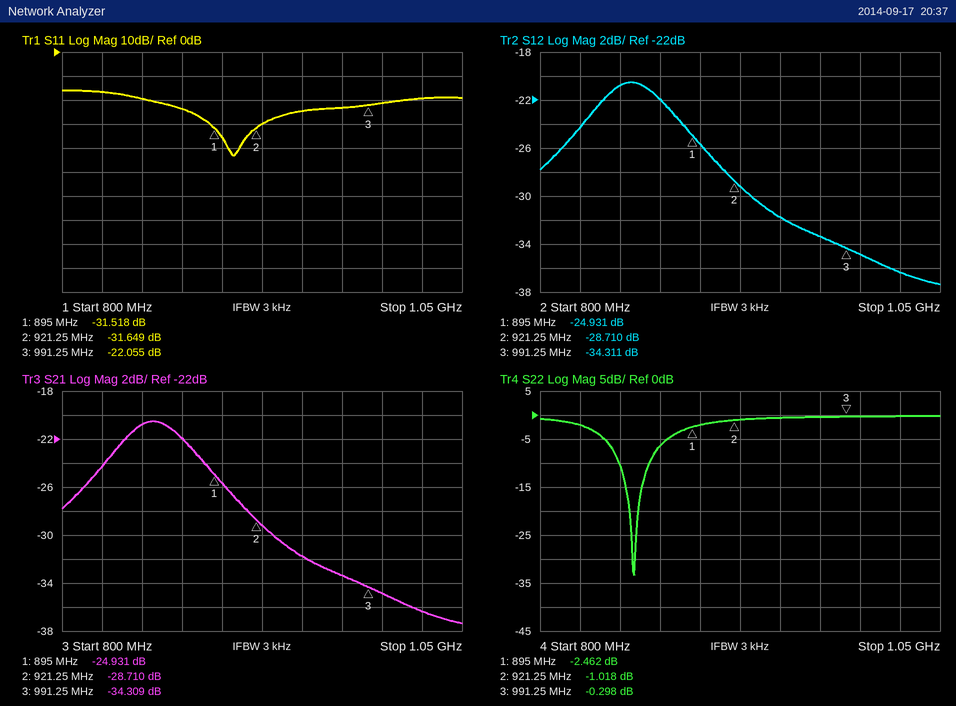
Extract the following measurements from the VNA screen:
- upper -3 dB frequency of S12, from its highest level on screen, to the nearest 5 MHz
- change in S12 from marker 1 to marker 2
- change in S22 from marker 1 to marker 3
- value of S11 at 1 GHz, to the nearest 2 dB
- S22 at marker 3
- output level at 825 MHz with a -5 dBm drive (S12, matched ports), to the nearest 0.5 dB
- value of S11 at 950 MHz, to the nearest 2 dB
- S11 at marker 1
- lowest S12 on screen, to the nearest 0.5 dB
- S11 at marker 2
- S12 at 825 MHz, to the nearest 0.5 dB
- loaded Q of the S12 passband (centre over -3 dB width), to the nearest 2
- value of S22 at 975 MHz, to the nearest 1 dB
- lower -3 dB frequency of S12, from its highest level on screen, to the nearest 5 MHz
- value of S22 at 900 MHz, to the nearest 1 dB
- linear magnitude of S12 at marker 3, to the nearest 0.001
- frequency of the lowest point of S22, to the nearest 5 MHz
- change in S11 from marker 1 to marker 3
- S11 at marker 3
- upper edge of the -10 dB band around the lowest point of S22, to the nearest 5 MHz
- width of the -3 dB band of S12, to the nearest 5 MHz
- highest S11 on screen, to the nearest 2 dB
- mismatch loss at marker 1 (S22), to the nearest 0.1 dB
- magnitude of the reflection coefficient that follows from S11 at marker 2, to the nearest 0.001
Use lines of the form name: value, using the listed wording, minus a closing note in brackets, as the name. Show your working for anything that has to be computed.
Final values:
upper -3 dB frequency of S12, from its highest level on screen, to the nearest 5 MHz: 885 MHz
change in S12 from marker 1 to marker 2: -28.71 − (-24.931) = -3.779 dB
change in S22 from marker 1 to marker 3: -0.298 − (-2.462) = 2.164 dB
value of S11 at 1 GHz, to the nearest 2 dB: -22 dB
S22 at marker 3: -0.298 dB
output level at 825 MHz with a -5 dBm drive (S12, matched ports), to the nearest 0.5 dB: -5 dBm + (-24.5 dB) = -29.5 dBm
value of S11 at 950 MHz, to the nearest 2 dB: -24 dB
S11 at marker 1: -31.518 dB
lowest S12 on screen, to the nearest 0.5 dB: -37.5 dB
S11 at marker 2: -31.649 dB
S12 at 825 MHz, to the nearest 0.5 dB: -24.5 dB
loaded Q of the S12 passband (centre over -3 dB width), to the nearest 2: 857.5 MHz / 55 MHz ≈ 16
value of S22 at 975 MHz, to the nearest 1 dB: 0 dB
lower -3 dB frequency of S12, from its highest level on screen, to the nearest 5 MHz: 830 MHz
value of S22 at 900 MHz, to the nearest 1 dB: -2 dB
linear magnitude of S12 at marker 3, to the nearest 0.001: 10^(-34.311/20) ≈ 0.019
frequency of the lowest point of S22, to the nearest 5 MHz: 860 MHz
change in S11 from marker 1 to marker 3: -22.055 − (-31.518) = 9.463 dB
S11 at marker 3: -22.055 dB
upper edge of the -10 dB band around the lowest point of S22, to the nearest 5 MHz: 870 MHz
width of the -3 dB band of S12, to the nearest 5 MHz: 885 MHz − 830 MHz = 55 MHz
highest S11 on screen, to the nearest 2 dB: -16 dB
mismatch loss at marker 1 (S22), to the nearest 0.1 dB: −10 log10(1 − 10^(-2.462/10)) ≈ 3.6 dB
magnitude of the reflection coefficient that follows from S11 at marker 2, to the nearest 0.001: 10^(-31.649/20) ≈ 0.026
